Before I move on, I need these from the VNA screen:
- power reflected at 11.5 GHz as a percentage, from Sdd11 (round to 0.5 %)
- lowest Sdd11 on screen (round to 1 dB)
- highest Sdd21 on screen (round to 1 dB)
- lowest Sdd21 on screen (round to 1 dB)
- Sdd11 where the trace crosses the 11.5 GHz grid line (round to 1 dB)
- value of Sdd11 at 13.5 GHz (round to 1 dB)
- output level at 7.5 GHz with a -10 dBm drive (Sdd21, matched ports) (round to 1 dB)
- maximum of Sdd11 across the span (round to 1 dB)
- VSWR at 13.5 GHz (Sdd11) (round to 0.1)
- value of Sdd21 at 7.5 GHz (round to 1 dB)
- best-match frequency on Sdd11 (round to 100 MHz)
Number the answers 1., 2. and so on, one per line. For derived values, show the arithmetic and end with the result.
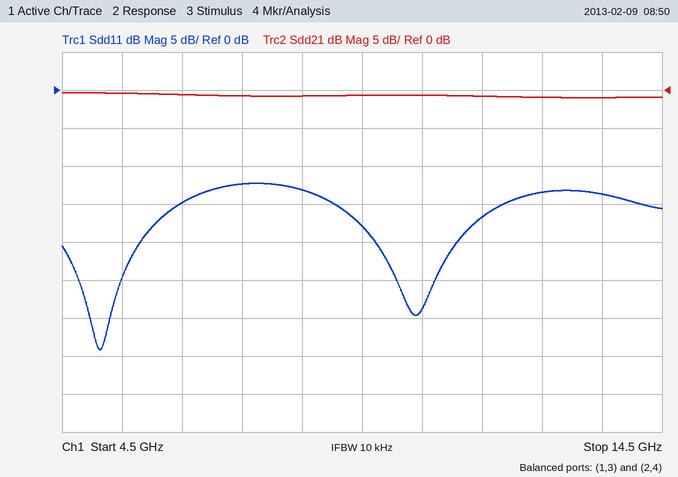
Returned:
1. 10^(-17/10) ≈ 2.0 %
2. -34 dB
3. 0 dB
4. -1 dB
5. -17 dB
6. -14 dB
7. -10 dBm + (-1 dB) = -11 dBm
8. -12 dB
9. |Γ| = 10^(-14/20) = 0.1995; VSWR = (1 + 0.1995)/(1 − 0.1995) ≈ 1.5
10. -1 dB
11. 5.1 GHz
